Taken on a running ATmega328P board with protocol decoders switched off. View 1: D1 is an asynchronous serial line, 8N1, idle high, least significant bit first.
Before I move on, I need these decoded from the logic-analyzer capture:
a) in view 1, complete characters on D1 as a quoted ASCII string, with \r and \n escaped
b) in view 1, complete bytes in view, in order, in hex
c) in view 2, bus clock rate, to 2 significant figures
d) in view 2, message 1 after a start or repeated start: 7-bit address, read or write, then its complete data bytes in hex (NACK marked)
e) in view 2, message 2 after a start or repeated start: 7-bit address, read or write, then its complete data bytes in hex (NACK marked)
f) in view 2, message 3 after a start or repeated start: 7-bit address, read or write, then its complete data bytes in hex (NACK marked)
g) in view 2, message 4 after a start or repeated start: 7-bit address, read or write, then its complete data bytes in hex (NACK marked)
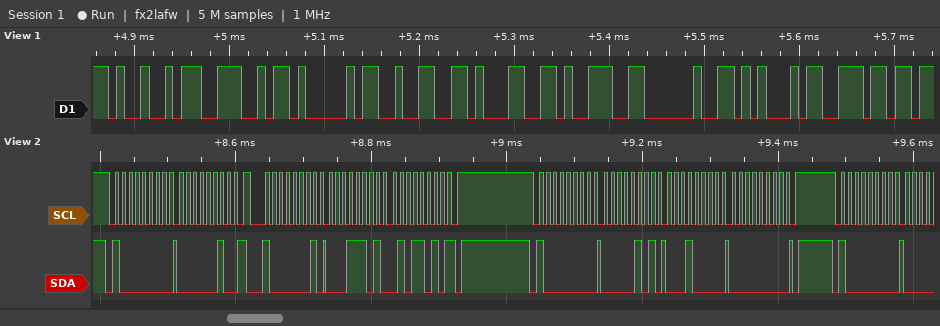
"INA219 En"
49 4E 41 32 31 39 20 45 6E
100 kHz
0x40 write: 02
0x40 read: 1D 5A NACK
0x40 write: 05 10 00
0x40 write
